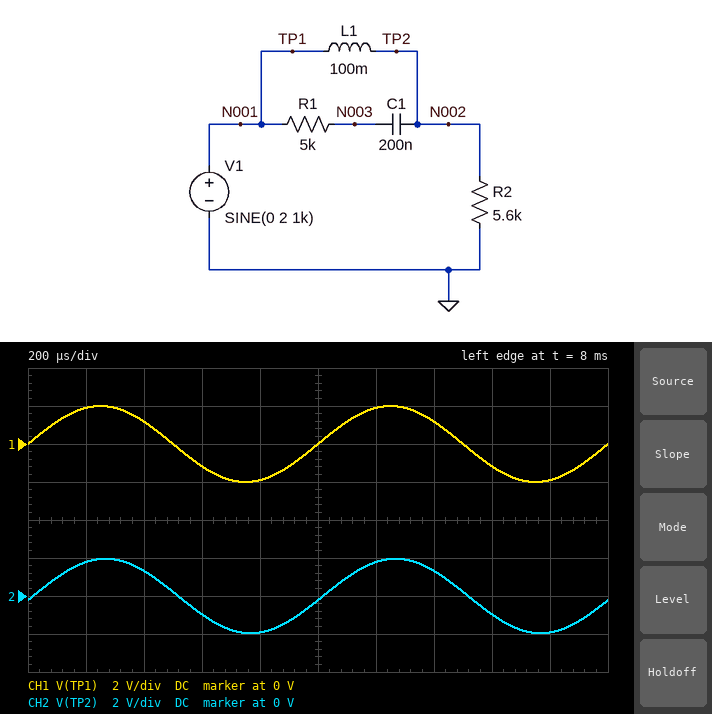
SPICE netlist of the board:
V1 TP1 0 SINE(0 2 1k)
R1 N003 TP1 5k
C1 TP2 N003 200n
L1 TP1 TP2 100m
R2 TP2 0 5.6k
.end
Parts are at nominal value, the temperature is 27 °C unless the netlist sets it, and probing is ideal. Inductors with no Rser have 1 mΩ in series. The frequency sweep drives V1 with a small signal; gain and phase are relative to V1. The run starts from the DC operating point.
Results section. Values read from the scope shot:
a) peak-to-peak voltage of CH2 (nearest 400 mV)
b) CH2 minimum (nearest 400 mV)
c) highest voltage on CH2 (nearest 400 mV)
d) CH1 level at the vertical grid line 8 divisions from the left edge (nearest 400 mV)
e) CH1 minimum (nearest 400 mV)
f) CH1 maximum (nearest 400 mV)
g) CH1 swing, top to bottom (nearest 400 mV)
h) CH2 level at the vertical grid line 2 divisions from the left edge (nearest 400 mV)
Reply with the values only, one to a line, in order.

4.0 V
-2.0 V
2.0 V
-1.2 V
-2.0 V
2.0 V
4.0 V
1.2 V
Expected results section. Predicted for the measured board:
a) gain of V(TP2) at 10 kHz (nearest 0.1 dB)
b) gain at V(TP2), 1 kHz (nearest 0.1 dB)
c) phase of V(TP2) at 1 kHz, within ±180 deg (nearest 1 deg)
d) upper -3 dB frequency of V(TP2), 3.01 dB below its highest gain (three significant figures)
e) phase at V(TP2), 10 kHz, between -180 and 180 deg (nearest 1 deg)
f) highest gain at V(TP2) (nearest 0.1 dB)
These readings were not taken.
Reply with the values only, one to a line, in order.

-4.2 dB
-0.2 dB
-6 deg
6.20 kHz
-16 deg
0 dB
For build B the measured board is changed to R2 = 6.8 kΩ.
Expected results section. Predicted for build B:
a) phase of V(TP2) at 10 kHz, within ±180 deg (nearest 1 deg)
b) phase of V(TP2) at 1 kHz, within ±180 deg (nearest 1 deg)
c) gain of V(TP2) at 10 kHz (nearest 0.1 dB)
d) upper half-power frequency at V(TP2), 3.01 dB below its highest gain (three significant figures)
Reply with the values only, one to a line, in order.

-14 deg
-5 deg
-3.5 dB
7.75 kHz
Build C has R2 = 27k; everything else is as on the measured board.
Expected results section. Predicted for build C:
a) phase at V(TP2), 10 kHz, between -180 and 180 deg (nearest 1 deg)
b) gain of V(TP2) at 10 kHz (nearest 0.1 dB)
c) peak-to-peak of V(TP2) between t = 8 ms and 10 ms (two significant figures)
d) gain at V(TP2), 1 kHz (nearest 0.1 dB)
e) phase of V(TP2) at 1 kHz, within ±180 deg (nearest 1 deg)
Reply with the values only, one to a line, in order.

-5 deg
-1.0 dB
4.0 V
0 dB
-1 deg
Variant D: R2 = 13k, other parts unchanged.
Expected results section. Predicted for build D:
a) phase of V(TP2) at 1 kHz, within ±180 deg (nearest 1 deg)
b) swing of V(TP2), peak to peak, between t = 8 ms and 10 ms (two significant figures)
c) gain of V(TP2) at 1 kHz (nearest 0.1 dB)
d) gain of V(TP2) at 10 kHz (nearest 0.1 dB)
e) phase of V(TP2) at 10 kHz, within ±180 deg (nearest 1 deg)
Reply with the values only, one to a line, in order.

-3 deg
4.0 V
-0.1 dB
-2.0 dB
-9 deg
